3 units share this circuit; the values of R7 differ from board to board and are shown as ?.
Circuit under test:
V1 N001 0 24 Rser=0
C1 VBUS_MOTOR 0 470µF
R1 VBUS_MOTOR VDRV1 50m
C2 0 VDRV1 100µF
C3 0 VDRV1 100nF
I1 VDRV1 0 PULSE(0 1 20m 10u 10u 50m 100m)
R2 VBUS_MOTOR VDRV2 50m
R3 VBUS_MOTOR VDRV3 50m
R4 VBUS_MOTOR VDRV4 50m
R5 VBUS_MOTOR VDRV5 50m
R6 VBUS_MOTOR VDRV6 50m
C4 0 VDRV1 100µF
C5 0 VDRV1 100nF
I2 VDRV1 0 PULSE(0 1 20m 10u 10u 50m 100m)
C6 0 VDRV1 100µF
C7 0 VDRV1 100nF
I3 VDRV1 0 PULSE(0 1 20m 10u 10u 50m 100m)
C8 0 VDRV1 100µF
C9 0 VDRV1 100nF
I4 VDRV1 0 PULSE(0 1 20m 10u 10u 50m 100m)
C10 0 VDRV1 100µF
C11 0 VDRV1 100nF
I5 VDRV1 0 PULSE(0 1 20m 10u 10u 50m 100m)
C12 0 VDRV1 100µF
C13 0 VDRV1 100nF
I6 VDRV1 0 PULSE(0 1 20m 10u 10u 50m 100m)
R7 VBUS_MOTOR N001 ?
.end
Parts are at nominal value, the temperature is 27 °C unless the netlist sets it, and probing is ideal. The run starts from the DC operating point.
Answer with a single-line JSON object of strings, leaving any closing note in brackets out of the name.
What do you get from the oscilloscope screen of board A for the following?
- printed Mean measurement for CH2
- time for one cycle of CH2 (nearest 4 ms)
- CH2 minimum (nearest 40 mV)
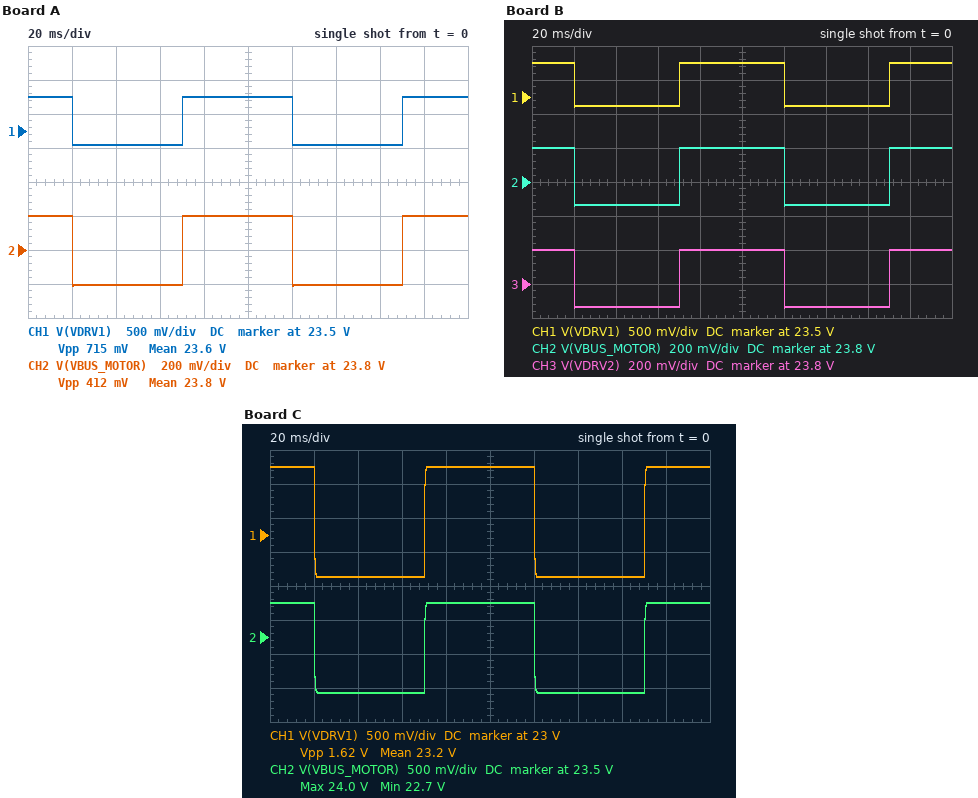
{"printed Mean measurement for CH2": "23.8 V", "time for one cycle of CH2": "100 ms", "CH2 minimum": "23.60 V"}
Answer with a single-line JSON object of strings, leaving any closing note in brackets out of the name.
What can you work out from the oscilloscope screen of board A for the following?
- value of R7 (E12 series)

{"value of R7": "0.068 Ω"}
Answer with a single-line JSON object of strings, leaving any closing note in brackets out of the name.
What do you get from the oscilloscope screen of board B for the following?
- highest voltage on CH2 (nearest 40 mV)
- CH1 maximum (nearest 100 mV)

{"highest voltage on CH2": "24.00 V", "CH1 maximum": "24.0 V"}
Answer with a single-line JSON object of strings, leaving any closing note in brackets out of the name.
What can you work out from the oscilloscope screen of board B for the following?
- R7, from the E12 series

{"R7, from the E12 series": "0.056 Ω"}
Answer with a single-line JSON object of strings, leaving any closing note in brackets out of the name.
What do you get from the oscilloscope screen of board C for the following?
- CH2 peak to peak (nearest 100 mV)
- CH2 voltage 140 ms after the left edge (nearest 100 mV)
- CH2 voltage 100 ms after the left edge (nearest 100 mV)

{"CH2 peak to peak": "1.3 V", "CH2 voltage 140 ms after the left edge": "22.7 V", "CH2 voltage 100 ms after the left edge": "24.0 V"}
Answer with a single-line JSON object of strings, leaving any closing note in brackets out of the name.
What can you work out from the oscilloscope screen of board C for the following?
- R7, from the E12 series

{"R7, from the E12 series": "0.22 Ω"}
